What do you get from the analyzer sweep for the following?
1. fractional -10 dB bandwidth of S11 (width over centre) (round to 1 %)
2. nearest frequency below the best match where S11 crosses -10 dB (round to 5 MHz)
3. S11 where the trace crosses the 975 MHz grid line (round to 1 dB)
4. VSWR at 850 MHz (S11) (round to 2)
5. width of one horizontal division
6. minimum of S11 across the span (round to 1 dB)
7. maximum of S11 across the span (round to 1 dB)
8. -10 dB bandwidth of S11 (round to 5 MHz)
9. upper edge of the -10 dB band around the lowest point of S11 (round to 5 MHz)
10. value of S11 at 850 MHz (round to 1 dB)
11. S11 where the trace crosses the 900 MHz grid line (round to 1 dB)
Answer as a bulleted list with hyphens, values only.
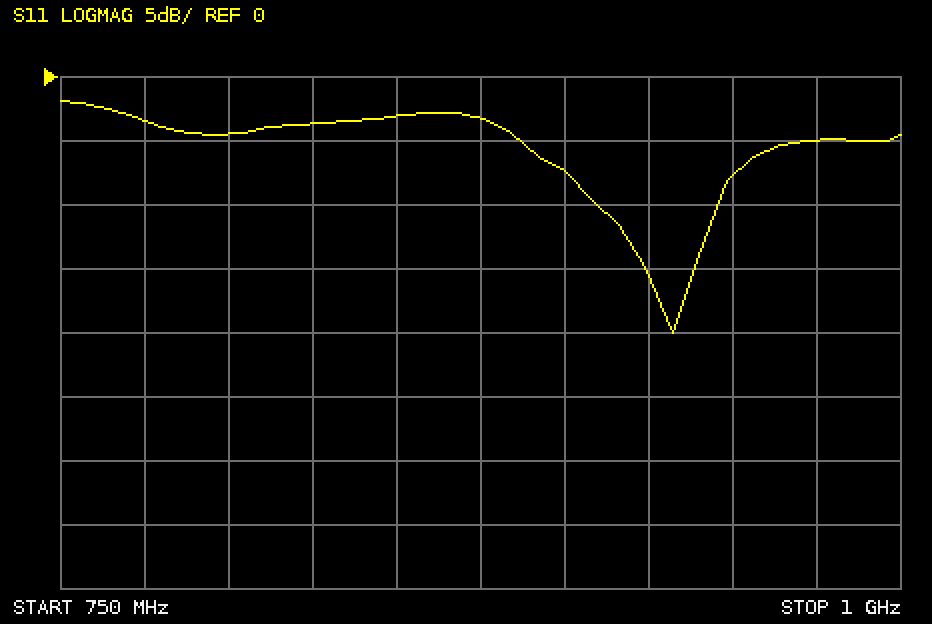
- 4 %
- 910 MHz
- -5 dB
- 6
- 25 MHz
- -20 dB
- -2 dB
- 35 MHz
- 945 MHz
- -3 dB
- -7 dB
